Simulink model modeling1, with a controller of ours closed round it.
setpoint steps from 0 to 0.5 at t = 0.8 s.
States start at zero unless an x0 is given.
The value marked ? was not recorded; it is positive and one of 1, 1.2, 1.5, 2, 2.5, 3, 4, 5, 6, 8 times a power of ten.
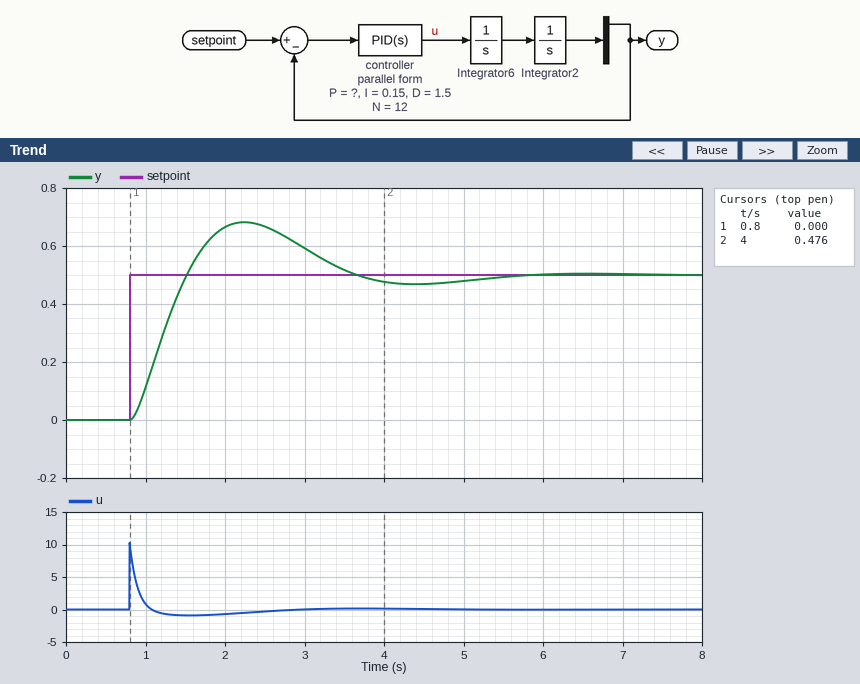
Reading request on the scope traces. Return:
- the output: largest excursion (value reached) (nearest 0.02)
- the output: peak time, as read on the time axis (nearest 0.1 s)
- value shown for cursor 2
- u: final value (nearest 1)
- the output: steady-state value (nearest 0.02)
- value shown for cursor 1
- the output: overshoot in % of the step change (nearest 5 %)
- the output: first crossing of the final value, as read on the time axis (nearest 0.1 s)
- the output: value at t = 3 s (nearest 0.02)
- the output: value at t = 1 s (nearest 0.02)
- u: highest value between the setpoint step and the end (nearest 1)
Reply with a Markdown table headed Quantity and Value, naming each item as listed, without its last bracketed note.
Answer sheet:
| Quantity | Value |
|---|---|
| the output: largest excursion (value reached) | 0.68 |
| the output: peak time, as read on the time axis | 2.2 s |
| value shown for cursor 2 | 0.476 |
| u: final value | 0 |
| the output: steady-state value | 0.50 |
| value shown for cursor 1 | 0.000 |
| the output: overshoot in % of the step change | 35 % |
| the output: first crossing of the final value, as read on the time axis | 1.5 s |
| the output: value at t = 3 s | 0.60 |
| the output: value at t = 1 s | 0.12 |
| u: highest value between the setpoint step and the end | 10 |
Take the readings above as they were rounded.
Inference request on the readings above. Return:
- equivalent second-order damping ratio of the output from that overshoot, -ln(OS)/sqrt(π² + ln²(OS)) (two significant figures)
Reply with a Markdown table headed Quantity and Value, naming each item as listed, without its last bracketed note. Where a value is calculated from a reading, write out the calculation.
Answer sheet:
| Quantity | Value |
|---|---|
| equivalent second-order damping ratio of the output from that overshoot, -ln(OS)/sqrt(π² + ln²(OS)) | ln(0.35) = -1.050; 1.050 / sqrt(9.870 + 1.102) = 0.32 |
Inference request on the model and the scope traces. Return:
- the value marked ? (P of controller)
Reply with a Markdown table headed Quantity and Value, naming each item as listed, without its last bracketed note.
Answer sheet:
| Quantity | Value |
|---|---|
| the value marked ? | 2.5 |
